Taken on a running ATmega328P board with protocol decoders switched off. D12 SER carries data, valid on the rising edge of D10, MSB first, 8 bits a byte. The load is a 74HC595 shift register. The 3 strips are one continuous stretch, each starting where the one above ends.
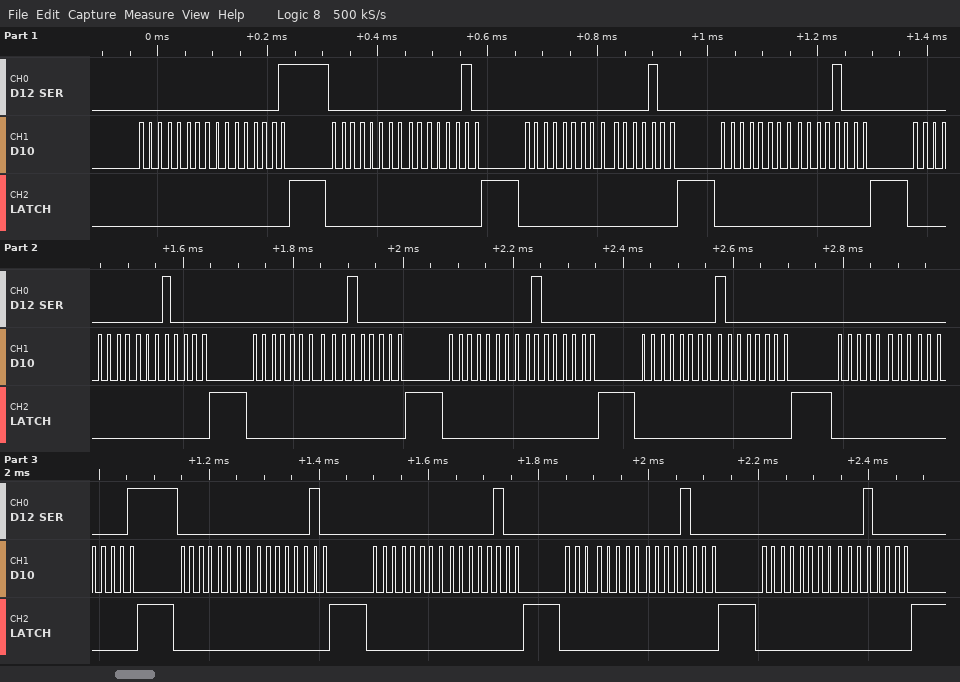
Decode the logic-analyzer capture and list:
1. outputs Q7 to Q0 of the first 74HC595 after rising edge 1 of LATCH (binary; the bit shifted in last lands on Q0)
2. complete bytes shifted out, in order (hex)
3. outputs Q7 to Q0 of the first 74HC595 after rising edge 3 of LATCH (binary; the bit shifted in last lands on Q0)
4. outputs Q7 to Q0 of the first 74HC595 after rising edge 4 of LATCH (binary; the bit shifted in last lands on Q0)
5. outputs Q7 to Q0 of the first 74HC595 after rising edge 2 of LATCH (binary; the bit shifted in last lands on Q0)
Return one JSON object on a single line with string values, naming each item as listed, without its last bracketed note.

{"outputs Q7 to Q0 of the first 74HC595 after rising edge 1 of LATCH": "00000001", "complete bytes shifted out, in order": "00 01 00 02 00 04 00 08 00 10 00 20 00 40 00 80 00 01 00 02 00 04 00 08 00 10", "outputs Q7 to Q0 of the first 74HC595 after rising edge 3 of LATCH": "00000100", "outputs Q7 to Q0 of the first 74HC595 after rising edge 4 of LATCH": "00001000", "outputs Q7 to Q0 of the first 74HC595 after rising edge 2 of LATCH": "00000010"}
